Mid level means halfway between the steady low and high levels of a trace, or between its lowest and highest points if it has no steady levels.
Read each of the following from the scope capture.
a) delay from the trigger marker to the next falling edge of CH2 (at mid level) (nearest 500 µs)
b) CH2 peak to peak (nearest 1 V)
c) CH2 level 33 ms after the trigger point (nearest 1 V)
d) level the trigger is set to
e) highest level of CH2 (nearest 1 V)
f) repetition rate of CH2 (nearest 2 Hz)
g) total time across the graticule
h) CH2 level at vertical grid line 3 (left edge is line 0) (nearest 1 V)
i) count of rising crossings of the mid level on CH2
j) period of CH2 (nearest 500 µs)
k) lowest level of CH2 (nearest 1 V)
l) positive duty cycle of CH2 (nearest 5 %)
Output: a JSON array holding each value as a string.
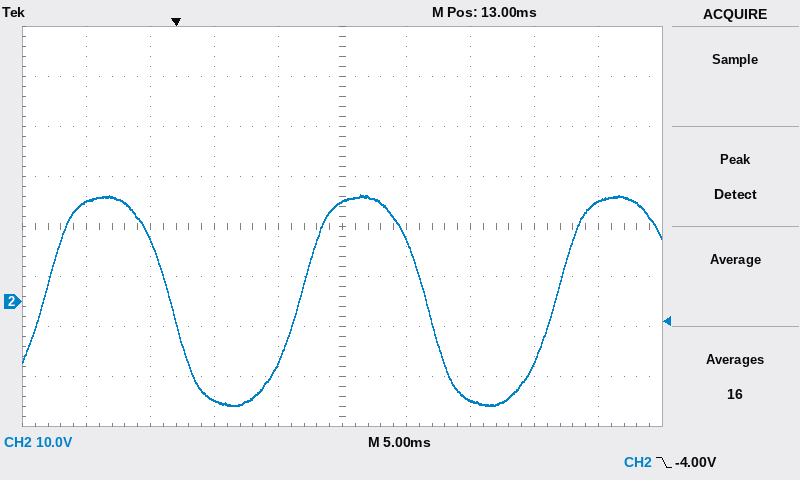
["19.5 ms", "42 V", "20 V", "-4.00 V", "21 V", "50 Hz", "50 ms", "-20 V", "3", "20.0 ms", "-21 V", "50 %"]
